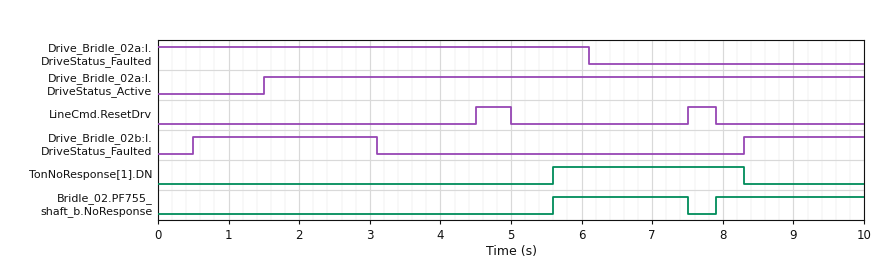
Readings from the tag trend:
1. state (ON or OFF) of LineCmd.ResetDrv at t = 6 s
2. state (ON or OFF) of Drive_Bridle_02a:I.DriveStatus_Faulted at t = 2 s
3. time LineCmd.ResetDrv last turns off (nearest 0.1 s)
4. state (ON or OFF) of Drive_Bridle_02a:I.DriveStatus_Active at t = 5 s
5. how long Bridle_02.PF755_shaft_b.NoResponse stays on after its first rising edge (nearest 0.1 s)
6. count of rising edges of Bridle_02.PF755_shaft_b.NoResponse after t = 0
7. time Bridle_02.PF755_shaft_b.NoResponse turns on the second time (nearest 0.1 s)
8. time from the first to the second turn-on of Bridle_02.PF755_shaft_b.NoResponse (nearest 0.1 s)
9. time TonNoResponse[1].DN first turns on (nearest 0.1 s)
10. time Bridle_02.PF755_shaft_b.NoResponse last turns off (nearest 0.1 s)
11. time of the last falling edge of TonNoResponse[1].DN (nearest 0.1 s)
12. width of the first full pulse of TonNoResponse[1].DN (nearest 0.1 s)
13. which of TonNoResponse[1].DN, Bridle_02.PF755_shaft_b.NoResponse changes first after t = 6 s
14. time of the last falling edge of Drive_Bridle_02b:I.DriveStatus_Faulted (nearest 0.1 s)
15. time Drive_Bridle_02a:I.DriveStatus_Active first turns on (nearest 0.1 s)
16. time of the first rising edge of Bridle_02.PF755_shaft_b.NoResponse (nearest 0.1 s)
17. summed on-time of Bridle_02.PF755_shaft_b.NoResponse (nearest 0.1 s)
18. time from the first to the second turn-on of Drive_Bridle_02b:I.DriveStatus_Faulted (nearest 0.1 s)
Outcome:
OFF
ON
7.9 s
ON
1.9 s
2
7.9 s
2.3 s
5.6 s
7.5 s
8.3 s
2.7 s
Bridle_02.PF755_shaft_b.NoResponse
3.1 s
1.5 s
5.6 s
4.0 s
7.8 s
